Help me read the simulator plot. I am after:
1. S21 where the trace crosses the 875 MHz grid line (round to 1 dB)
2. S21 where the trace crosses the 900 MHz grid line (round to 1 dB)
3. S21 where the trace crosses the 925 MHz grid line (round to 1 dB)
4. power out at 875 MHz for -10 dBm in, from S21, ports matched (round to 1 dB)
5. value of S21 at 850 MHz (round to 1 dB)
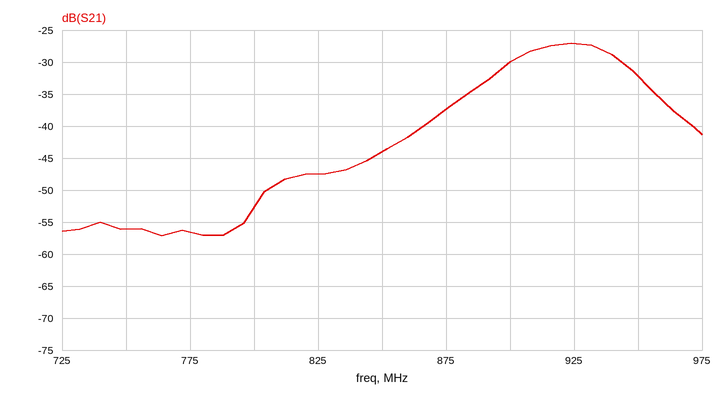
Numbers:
-37 dB
-30 dB
-27 dB
-47 dBm
-44 dB
